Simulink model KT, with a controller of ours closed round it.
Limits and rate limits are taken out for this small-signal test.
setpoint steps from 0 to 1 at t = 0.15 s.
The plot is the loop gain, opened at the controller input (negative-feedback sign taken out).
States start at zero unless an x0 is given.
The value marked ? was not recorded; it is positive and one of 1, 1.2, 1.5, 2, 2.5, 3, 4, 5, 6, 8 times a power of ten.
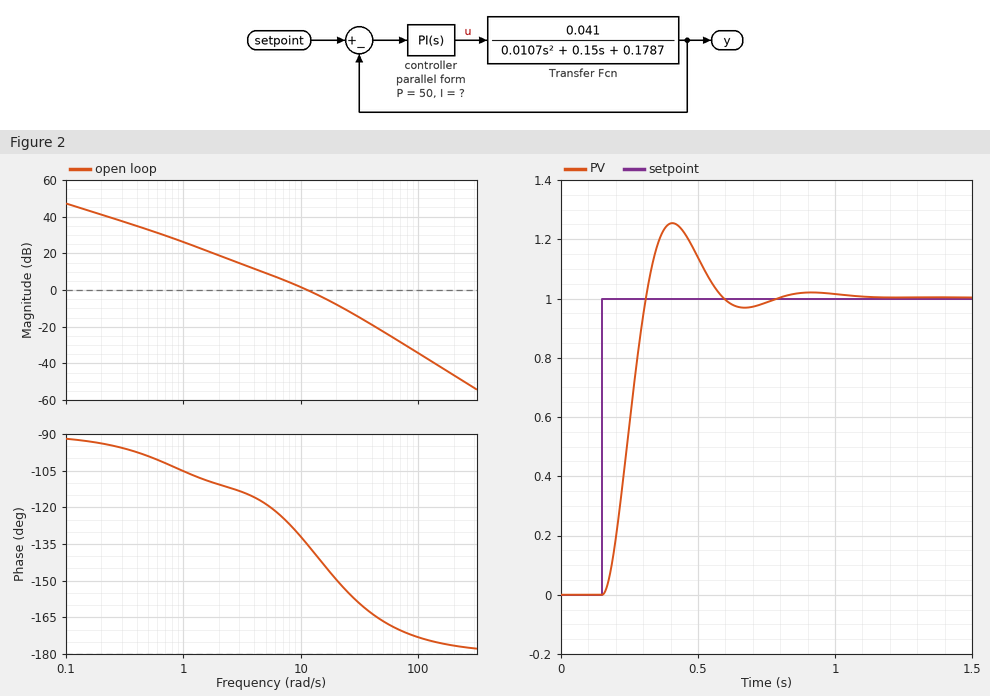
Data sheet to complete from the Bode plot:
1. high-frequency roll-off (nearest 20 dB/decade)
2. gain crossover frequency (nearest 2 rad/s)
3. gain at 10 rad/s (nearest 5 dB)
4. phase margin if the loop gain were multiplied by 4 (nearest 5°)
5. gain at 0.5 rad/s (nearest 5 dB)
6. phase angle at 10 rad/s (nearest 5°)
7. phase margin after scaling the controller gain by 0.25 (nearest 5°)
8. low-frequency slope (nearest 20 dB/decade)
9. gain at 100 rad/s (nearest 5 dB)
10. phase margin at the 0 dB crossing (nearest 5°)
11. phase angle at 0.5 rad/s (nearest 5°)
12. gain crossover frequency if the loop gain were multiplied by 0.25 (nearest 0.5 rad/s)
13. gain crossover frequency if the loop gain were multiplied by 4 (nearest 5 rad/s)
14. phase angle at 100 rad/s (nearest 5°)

-40 dB/decade
12 rad/s
0 dB
25°
35 dB
-130°
65°
-20 dB/decade
-35 dB
45°
-100°
4.0 rad/s
25 rad/s
-175°
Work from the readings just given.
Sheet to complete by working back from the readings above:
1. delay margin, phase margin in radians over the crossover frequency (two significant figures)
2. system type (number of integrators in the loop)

0.065 s
1
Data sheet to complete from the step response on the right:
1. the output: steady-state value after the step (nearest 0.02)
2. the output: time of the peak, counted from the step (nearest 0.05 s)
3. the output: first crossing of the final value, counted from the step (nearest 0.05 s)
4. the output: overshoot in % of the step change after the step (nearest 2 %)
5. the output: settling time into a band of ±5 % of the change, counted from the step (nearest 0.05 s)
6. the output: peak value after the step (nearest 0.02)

1.00
0.25 s
0.15 s
26 %
0.40 s
1.26
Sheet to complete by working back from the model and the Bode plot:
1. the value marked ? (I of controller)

100
